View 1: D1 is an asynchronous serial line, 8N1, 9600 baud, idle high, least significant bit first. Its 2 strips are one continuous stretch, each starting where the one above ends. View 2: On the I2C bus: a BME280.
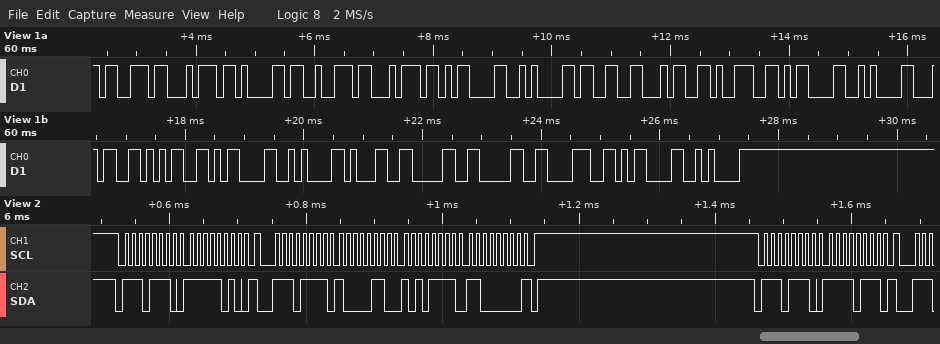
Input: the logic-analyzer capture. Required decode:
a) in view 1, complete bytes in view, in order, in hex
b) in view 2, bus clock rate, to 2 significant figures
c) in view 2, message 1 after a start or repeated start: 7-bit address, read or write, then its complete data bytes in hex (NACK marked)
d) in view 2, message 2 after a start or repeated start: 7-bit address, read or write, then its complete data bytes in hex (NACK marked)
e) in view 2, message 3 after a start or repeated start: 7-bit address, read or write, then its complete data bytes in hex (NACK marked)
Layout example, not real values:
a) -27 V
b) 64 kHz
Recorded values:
a) 73 74 61 72 74 0D 0A 33 34 39 0D 0A 34 35 0D 0A 31 30 30 38 0D 0A
b) 100 kHz
c) 0x77 write: FA
d) 0x77 read: 86 AF C0 NACK
e) 0x77 write: F7
